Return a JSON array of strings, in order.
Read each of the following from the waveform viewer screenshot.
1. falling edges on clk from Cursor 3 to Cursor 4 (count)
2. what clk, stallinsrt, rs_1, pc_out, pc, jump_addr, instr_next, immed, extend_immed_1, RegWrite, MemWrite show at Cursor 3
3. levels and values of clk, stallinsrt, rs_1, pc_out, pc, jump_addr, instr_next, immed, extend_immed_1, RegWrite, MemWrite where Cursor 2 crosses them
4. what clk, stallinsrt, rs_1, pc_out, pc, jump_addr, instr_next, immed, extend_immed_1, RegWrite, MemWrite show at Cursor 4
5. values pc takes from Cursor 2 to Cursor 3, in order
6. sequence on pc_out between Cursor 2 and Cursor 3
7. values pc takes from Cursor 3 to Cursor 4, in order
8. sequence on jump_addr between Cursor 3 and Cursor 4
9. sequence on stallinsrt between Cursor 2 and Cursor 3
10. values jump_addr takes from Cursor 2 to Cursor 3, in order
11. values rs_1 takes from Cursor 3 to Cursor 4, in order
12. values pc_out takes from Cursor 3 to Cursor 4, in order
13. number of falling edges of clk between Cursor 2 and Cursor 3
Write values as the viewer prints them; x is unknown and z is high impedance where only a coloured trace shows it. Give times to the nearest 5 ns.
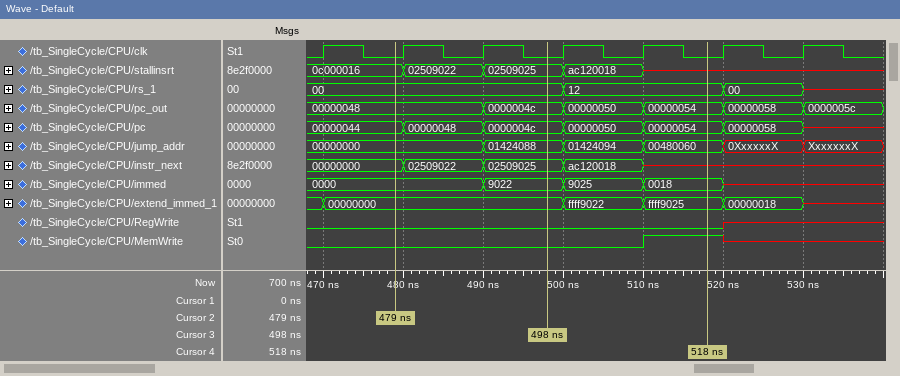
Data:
["2", "clk=0, stallinsrt=02509025, rs_1=00, pc_out=0000004c, pc=0000004c, jump_addr=01424088, instr_next=02509025, immed=9022, extend_immed_1=00000000, RegWrite=0, MemWrite=0", "clk=0, stallinsrt=0c000016, rs_1=00, pc_out=00000048, pc=00000044, jump_addr=00000000, instr_next=00000000, immed=0000, extend_immed_1=00000000, RegWrite=0, MemWrite=0", "clk=0, stallinsrt=x, rs_1=12, pc_out=00000054, pc=00000054, jump_addr=00480060, instr_next=x, immed=0018, extend_immed_1=ffff9025, RegWrite=0, MemWrite=1", "00000044, 00000048, 0000004c", "00000048, 0000004c", "0000004c, 00000050, 00000054", "01424088, 01424094, 00480060", "0c000016, 02509022, 02509025", "00000000, 01424088", "00, 12", "0000004c, 00000050, 00000054", "2"]
